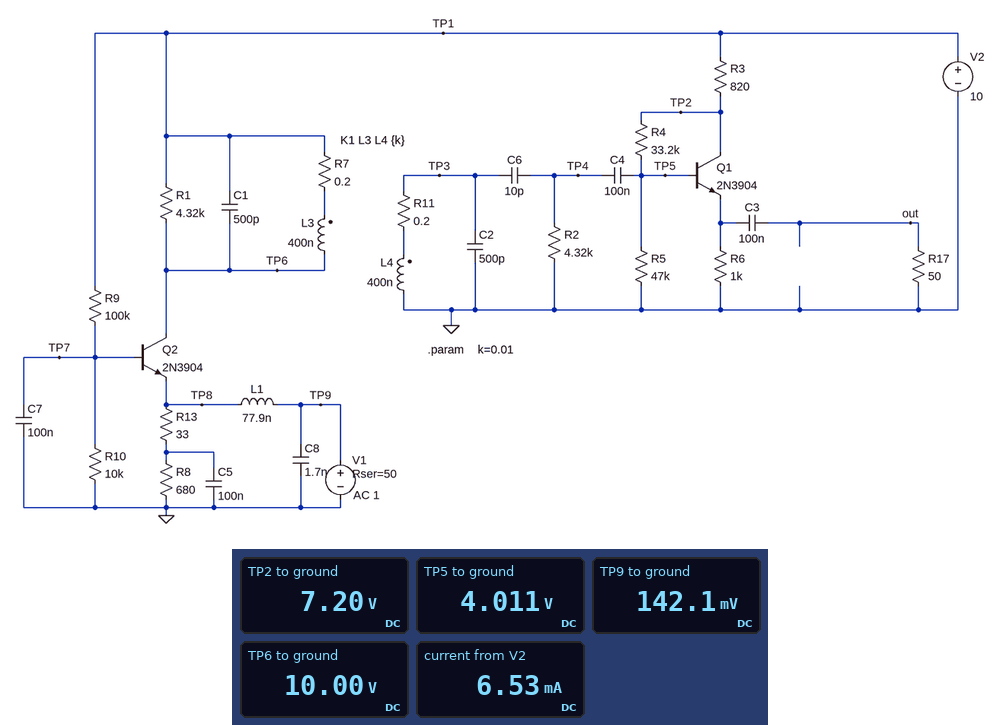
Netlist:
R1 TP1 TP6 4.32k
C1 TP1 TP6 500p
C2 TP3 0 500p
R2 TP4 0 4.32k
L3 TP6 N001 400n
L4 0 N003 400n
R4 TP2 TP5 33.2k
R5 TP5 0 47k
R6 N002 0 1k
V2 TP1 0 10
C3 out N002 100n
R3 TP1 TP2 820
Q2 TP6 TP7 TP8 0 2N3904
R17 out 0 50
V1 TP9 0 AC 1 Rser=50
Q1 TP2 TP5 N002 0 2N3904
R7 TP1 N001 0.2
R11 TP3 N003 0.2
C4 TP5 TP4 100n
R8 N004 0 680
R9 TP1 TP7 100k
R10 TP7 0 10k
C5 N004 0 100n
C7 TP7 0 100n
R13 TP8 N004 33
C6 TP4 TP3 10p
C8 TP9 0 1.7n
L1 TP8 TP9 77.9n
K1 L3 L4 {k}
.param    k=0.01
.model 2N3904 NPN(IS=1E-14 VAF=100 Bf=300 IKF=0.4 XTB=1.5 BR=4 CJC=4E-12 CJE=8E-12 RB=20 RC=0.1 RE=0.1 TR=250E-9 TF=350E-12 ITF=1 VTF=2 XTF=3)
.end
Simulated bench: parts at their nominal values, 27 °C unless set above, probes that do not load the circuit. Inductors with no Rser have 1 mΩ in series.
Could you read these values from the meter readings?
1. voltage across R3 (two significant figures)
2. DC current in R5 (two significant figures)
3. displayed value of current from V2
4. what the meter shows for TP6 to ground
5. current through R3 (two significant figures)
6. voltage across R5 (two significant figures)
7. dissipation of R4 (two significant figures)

2.8 V
85 µA
6.53 mA
10.00 V
3.4 mA
4.0 V
310 µW
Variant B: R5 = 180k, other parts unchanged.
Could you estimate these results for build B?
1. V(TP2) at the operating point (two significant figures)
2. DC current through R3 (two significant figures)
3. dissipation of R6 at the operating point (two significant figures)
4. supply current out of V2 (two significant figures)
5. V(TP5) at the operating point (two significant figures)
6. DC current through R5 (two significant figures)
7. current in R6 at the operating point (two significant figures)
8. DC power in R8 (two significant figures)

6.4 V
4.4 mA
19 mW
7.5 mA
5.0 V
28 µA
4.3 mA
27 µW
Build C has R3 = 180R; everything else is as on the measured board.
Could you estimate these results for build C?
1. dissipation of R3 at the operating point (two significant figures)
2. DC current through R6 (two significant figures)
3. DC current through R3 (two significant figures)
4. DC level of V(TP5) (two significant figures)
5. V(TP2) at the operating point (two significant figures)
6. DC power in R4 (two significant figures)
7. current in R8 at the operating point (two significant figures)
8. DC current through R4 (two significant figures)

3.7 mW
4.4 mA
4.5 mA
5.1 V
9.2 V
500 µW
200 µA
120 µA
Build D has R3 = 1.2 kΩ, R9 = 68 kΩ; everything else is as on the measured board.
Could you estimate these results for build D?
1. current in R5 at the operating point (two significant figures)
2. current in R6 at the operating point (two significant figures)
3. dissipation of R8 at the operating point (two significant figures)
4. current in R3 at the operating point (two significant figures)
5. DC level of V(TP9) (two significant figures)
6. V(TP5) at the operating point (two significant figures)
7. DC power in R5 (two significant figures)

76 µA
2.9 mA
180 µW
3.0 mA
360 mV
3.6 V
270 µW
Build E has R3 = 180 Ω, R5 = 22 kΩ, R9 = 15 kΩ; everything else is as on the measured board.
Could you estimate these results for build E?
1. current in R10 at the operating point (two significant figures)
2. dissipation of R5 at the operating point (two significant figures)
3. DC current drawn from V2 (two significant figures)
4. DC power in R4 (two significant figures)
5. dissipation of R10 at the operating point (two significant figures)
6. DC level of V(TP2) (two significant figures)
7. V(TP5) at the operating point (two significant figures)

300 µA
600 µW
51 mA
1.0 mW
900 µW
9.4 V
3.6 V
